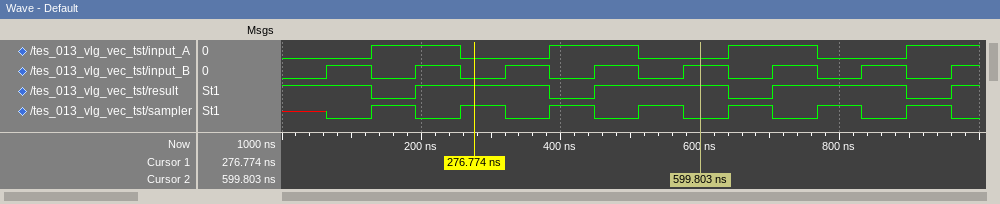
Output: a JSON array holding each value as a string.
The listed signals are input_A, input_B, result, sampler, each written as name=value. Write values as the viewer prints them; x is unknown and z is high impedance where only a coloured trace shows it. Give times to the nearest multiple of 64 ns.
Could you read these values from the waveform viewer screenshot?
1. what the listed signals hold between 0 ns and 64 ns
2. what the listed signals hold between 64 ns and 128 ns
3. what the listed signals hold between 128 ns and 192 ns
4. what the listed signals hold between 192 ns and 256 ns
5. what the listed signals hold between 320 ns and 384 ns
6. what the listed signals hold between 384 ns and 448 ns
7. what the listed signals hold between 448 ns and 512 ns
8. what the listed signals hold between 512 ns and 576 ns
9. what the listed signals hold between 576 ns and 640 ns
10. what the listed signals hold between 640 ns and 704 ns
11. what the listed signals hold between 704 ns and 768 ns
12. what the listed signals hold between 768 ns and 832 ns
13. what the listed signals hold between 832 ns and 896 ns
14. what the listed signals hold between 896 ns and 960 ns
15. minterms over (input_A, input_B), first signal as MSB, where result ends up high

["input_A=0, input_B=0, result=1, sampler=x", "input_A=0, input_B=1, result=1, sampler=0", "input_A=1, input_B=0, result=0, sampler=1", "input_A=1, input_B=1, result=1, sampler=0", "input_A=0, input_B=1, result=1, sampler=0", "input_A=1, input_B=0, result=0, sampler=1", "input_A=1, input_B=1, result=1, sampler=0", "input_A=0, input_B=0, result=1, sampler=1", "input_A=0, input_B=1, result=1, sampler=0", "input_A=1, input_B=0, result=0, sampler=1", "input_A=1, input_B=1, result=1, sampler=0", "input_A=0, input_B=0, result=1, sampler=1", "input_A=0, input_B=1, result=1, sampler=0", "input_A=1, input_B=0, result=0, sampler=1", "0, 1, 3"]
